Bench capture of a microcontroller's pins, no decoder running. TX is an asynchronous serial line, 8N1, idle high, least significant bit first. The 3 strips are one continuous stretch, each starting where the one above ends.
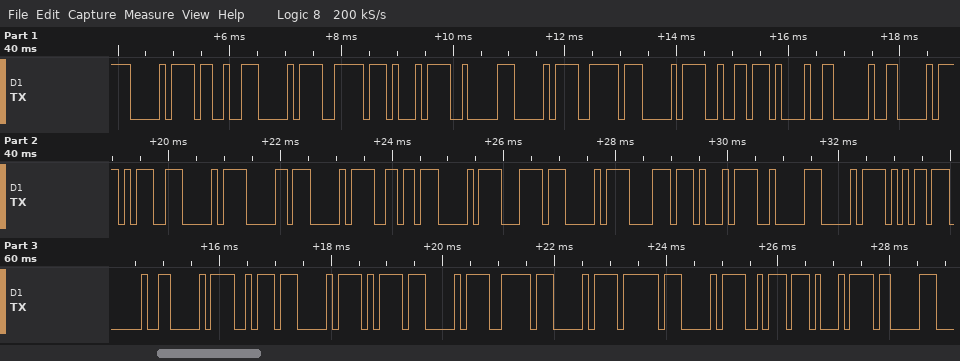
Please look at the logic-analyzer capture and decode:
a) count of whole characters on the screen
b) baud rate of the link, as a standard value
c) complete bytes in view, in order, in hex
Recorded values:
39
9600 baud
D0 93 D0 BE D1 82 D0 BE D0 B2 21 20 D0 9D D0 B0 D0 B6 D0 BC D0 B8 D1 82 D0 B5 20 D0 BA D0 BD D0 BE D0 BF D0 BA D1 83
